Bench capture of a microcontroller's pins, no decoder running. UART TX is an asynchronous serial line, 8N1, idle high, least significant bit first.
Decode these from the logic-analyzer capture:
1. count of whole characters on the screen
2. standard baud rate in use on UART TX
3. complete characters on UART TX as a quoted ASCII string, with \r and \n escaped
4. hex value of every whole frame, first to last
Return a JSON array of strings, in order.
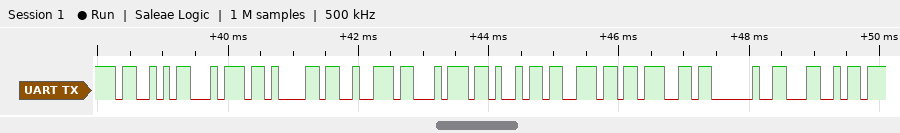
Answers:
["10", "9600 baud", "\"Starting L\"", "53 74 61 72 74 69 6E 67 20 4C"]
